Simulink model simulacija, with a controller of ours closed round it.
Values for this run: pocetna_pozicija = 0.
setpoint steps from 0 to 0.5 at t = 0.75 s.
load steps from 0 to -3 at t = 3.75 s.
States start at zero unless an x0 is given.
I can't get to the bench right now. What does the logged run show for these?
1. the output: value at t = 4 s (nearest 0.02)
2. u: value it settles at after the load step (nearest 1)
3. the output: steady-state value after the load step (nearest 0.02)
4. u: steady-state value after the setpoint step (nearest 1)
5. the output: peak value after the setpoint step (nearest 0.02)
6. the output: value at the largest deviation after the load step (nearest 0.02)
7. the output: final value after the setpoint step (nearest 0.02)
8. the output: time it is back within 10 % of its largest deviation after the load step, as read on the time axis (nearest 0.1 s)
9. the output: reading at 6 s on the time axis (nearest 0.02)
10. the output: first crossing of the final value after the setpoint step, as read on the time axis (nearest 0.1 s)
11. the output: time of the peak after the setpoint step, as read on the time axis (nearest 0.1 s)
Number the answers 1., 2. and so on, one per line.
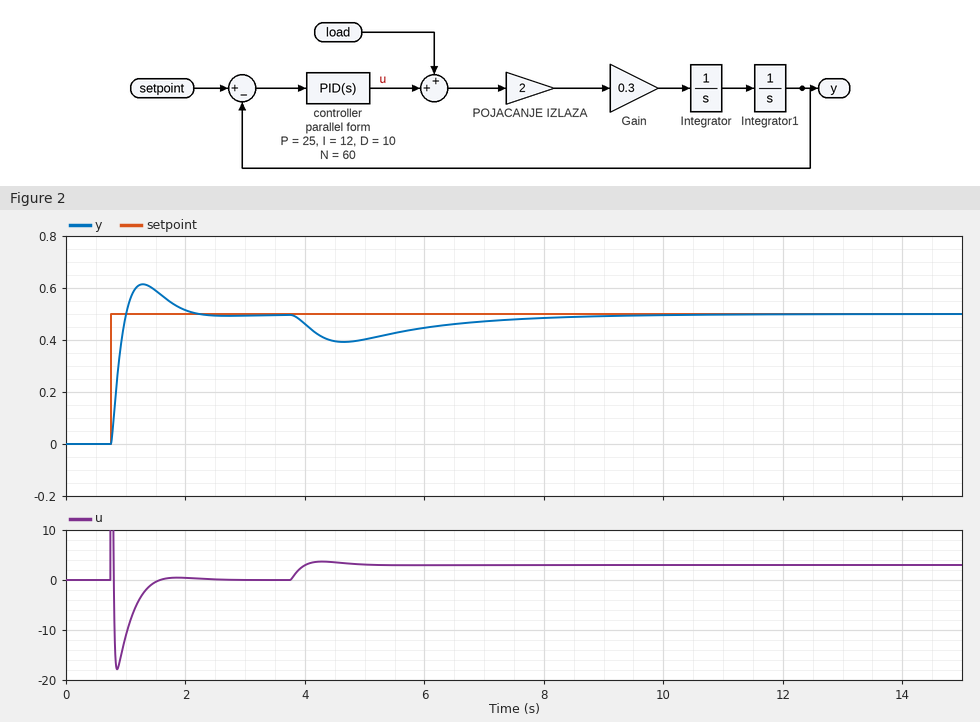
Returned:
1. 0.46
2. 3
3. 0.50
4. 0
5. 0.62
6. 0.40
7. 0.50
8. 8.6 s
9. 0.44
10. 1.0 s
11. 1.3 s
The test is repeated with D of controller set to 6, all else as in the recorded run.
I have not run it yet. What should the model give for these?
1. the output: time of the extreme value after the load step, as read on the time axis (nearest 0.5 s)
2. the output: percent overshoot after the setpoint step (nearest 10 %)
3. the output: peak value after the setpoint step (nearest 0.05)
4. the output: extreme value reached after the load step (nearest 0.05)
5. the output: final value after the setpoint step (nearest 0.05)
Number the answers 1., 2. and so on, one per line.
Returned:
1. 4.5 s
2. 40 %
3. 0.70
4. 0.35
5. 0.50
